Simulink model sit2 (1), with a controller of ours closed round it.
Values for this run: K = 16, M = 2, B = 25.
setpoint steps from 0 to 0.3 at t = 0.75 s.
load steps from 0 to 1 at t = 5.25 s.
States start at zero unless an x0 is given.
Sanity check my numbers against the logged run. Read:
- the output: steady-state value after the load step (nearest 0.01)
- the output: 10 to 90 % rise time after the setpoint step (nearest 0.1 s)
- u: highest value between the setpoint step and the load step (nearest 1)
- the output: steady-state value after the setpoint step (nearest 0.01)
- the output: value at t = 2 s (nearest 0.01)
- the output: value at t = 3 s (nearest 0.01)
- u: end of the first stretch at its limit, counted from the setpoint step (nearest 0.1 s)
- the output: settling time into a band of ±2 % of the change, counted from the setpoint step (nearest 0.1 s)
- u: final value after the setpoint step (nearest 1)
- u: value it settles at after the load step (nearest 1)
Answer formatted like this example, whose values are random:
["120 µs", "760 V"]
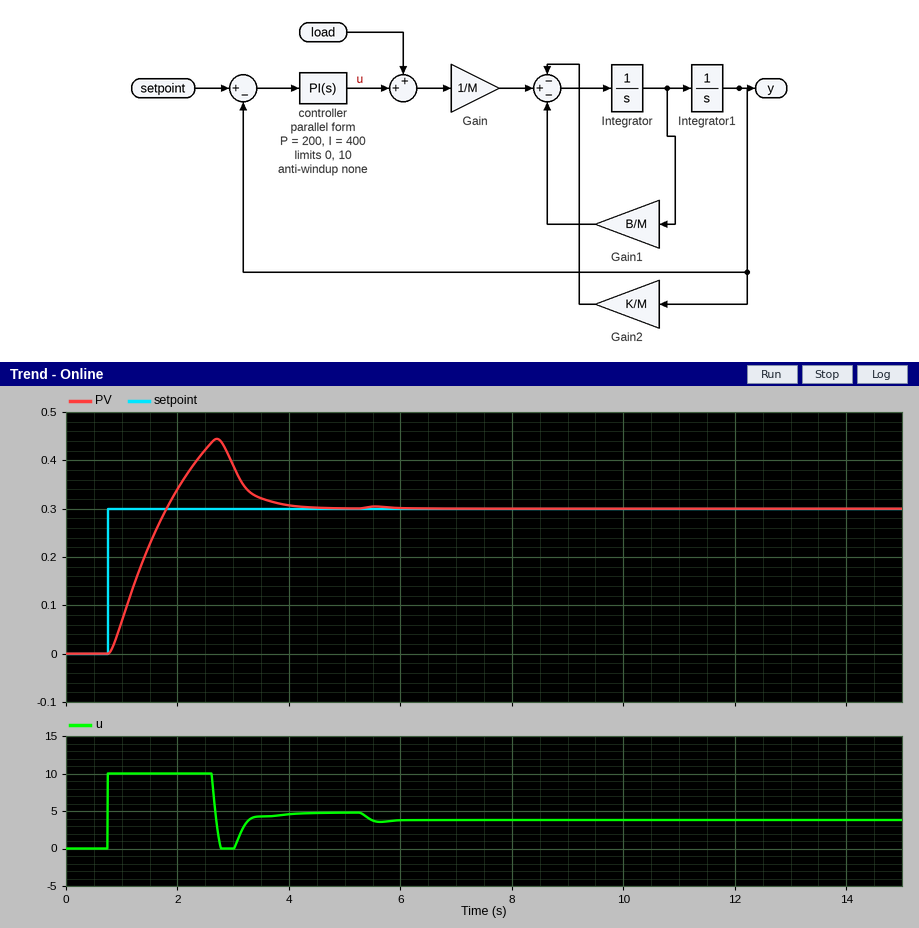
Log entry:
["0.30", "0.8 s", "10", "0.30", "0.34", "0.39", "1.9 s", "3.3 s", "5", "4"]
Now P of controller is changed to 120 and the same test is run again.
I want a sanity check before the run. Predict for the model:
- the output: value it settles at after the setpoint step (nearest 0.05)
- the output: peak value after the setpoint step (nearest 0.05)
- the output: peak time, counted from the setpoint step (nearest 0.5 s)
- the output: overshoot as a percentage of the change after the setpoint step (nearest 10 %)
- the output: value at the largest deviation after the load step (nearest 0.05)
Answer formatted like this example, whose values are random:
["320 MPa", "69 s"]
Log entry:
["0.30", "0.45", "2.0 s", "50 %", "0.30"]
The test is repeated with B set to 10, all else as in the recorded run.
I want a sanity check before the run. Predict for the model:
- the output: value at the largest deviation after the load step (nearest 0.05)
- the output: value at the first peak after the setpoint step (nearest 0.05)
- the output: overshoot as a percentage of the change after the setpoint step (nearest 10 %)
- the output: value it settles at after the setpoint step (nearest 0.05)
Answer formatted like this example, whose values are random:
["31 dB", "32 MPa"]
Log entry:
["0.30", "0.45", "50 %", "0.30"]
